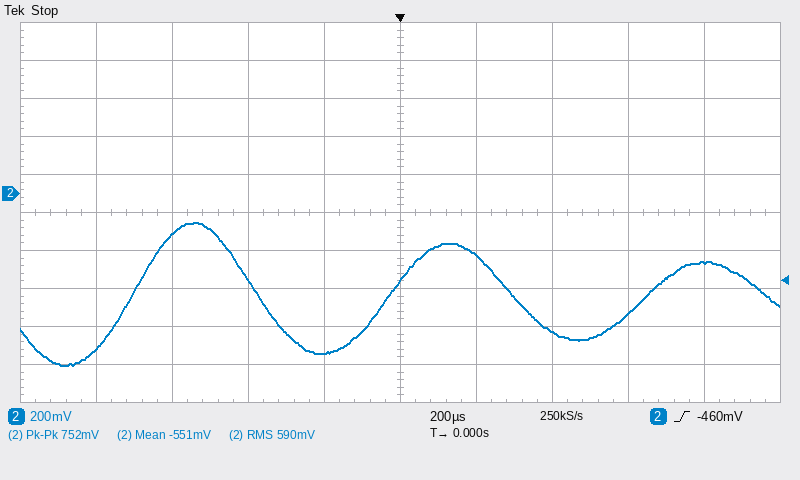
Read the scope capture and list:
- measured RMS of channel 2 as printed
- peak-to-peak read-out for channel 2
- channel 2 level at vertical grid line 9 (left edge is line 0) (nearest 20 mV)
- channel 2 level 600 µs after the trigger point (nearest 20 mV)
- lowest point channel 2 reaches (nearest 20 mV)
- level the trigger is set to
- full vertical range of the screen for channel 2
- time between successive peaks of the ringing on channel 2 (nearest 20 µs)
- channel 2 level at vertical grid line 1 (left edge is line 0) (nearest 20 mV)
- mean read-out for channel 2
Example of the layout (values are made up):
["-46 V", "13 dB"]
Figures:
["590 mV", "752 mV", "-360 mV", "-640 mV", "-900 mV", "-460 mV", "2 V", "680 µs", "-820 mV", "-551 mV"]
